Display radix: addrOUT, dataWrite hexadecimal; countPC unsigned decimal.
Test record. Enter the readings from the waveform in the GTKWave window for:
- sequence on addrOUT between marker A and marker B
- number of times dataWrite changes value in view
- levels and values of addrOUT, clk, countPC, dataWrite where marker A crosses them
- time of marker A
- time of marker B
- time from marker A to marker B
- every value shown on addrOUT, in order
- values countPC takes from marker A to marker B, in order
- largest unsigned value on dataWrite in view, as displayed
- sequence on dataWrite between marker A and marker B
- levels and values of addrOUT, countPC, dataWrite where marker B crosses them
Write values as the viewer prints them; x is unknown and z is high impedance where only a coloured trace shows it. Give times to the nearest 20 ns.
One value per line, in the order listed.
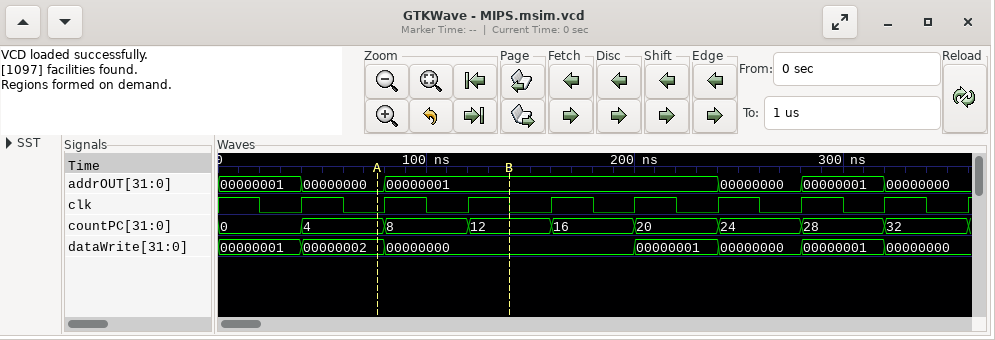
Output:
00000000, 00000001
6
addrOUT=00000000, clk=0, countPC=4, dataWrite=00000002
80 ns
140 ns
60 ns
00000001, 00000000, 00000001, 00000000, 00000001, 00000000
4, 8, 12
00000002
00000002, 00000000
addrOUT=00000001, countPC=12, dataWrite=00000000
